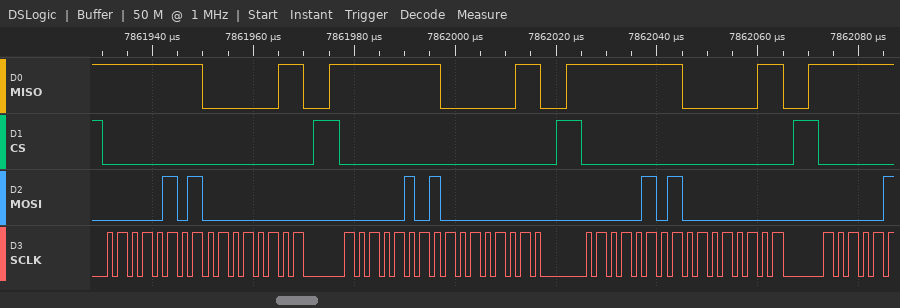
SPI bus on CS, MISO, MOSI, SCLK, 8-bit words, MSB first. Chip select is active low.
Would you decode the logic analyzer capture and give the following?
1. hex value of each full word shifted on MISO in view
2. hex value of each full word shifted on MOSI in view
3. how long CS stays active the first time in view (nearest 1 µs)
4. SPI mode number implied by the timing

FF, 03, FF, 03, FF, 03
05, 00, 05, 00, 05, 00
42 µs
0
